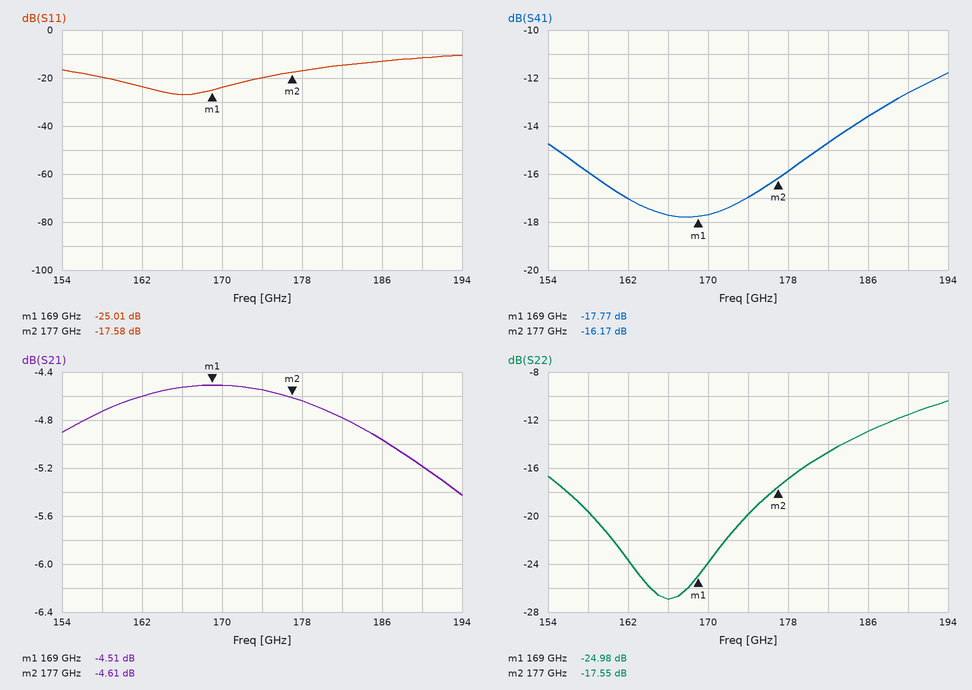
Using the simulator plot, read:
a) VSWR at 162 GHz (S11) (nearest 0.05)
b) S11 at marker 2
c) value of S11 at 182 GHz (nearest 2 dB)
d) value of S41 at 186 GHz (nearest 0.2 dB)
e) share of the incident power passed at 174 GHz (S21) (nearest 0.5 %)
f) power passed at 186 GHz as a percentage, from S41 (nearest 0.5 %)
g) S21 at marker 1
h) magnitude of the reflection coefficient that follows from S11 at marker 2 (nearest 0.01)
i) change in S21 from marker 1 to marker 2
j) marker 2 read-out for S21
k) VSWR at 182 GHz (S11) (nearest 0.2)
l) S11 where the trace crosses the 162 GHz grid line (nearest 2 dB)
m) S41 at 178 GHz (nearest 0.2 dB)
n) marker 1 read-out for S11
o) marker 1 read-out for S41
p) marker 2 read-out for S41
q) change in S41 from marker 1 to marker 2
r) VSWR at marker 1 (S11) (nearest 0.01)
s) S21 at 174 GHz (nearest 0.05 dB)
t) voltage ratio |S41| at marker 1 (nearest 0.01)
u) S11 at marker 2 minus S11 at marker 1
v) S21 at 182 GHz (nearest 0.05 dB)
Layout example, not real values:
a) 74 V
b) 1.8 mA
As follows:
a) 1.15
b) -17.58 dB
c) -14 dB
d) -13.6 dB
e) 35.0 %
f) 4.5 %
g) -4.51 dB
h) 0.13
i) -0.10 dB
j) -4.61 dB
k) 1.4
l) -24 dB
m) -15.8 dB
n) -25.01 dB
o) -17.77 dB
p) -16.17 dB
q) 1.60 dB
r) 1.12
s) -4.55 dB
t) 0.13
u) 7.43 dB
v) -4.80 dB
